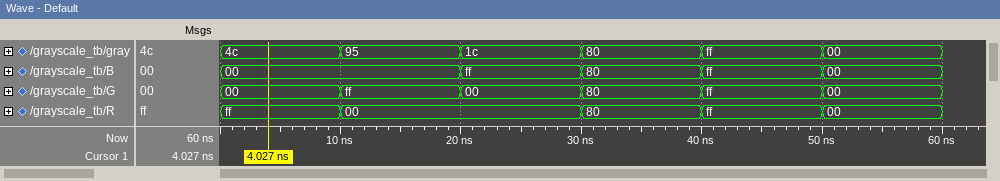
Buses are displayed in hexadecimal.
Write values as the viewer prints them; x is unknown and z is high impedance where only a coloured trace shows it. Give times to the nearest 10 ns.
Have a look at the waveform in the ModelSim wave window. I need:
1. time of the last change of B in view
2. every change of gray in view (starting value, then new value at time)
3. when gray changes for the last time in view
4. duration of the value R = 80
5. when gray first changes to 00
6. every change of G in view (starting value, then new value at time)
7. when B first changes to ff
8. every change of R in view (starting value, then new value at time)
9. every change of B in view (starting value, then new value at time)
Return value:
50 ns
4c, 95 at 10 ns, 1c at 20 ns, 80 at 30 ns, ff at 40 ns, 00 at 50 ns
50 ns
10 ns
50 ns
00, ff at 10 ns, 00 at 20 ns, 80 at 30 ns, ff at 40 ns, 00 at 50 ns
20 ns
ff, 00 at 10 ns, 80 at 30 ns, ff at 40 ns, 00 at 50 ns
00, ff at 20 ns, 80 at 30 ns, ff at 40 ns, 00 at 50 ns
